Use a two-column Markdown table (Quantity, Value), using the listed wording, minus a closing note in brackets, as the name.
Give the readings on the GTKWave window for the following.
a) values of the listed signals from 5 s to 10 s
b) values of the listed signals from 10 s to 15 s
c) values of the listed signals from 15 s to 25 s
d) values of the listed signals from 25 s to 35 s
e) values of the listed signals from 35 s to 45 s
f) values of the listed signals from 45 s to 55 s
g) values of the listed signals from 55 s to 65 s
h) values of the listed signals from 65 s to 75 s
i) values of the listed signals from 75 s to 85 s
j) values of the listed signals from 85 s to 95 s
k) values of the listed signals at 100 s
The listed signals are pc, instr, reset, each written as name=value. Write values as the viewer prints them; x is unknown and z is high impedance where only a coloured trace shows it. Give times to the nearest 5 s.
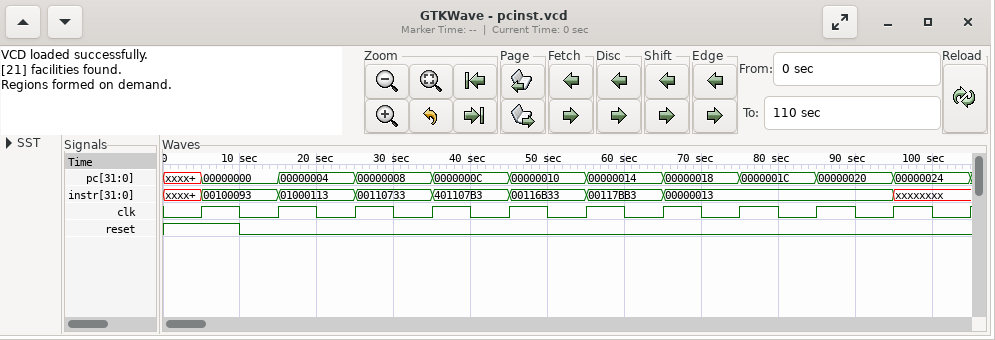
| Quantity | Value |
|---|---|
| values of the listed signals from 5 s to 10 s | pc=00000000, instr=00100093, reset=1 |
| values of the listed signals from 10 s to 15 s | pc=00000000, instr=00100093, reset=0 |
| values of the listed signals from 15 s to 25 s | pc=00000004, instr=01000113, reset=0 |
| values of the listed signals from 25 s to 35 s | pc=00000008, instr=00110733, reset=0 |
| values of the listed signals from 35 s to 45 s | pc=0000000C, instr=401107B3, reset=0 |
| values of the listed signals from 45 s to 55 s | pc=00000010, instr=00116B33, reset=0 |
| values of the listed signals from 55 s to 65 s | pc=00000014, instr=00117BB3, reset=0 |
| values of the listed signals from 65 s to 75 s | pc=00000018, instr=00000013, reset=0 |
| values of the listed signals from 75 s to 85 s | pc=0000001C, instr=00000013, reset=0 |
| values of the listed signals from 85 s to 95 s | pc=00000020, instr=00000013, reset=0 |
| values of the listed signals at 100 s | pc=00000024, instr=xxxxxxxx, reset=0 |
